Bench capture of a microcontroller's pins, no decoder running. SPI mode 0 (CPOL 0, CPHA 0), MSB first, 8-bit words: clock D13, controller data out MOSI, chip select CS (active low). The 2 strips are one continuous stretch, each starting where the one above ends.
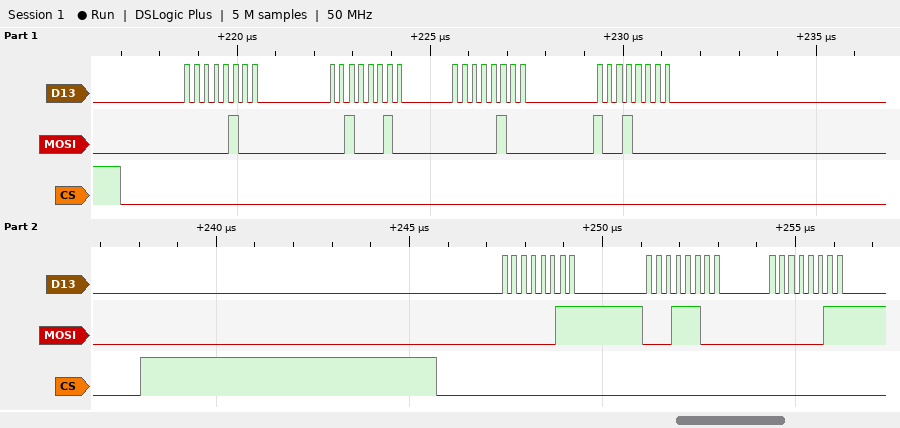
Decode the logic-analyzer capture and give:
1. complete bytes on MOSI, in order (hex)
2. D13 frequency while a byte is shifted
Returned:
04 22 04 90 03 1C 03
4 MHz
